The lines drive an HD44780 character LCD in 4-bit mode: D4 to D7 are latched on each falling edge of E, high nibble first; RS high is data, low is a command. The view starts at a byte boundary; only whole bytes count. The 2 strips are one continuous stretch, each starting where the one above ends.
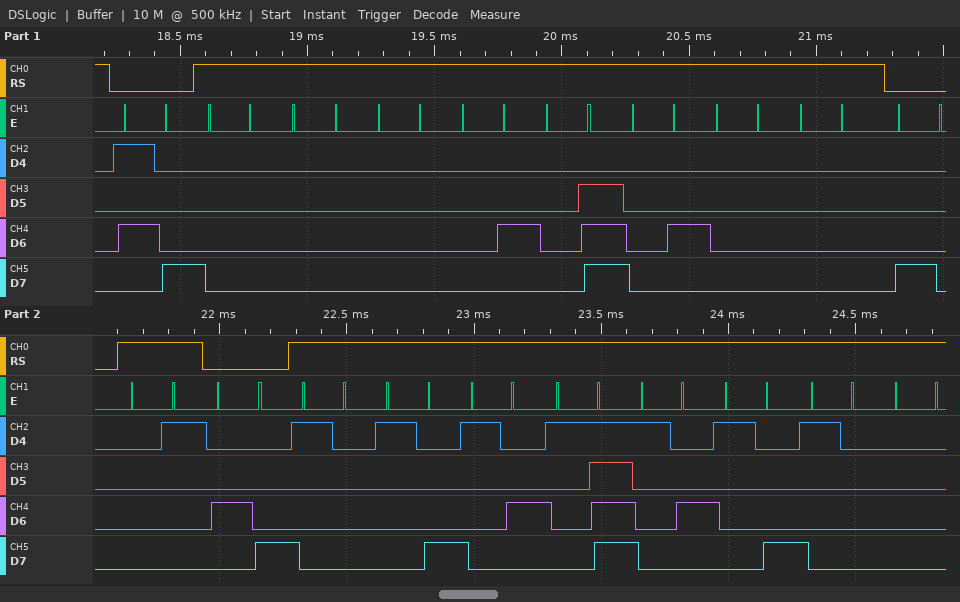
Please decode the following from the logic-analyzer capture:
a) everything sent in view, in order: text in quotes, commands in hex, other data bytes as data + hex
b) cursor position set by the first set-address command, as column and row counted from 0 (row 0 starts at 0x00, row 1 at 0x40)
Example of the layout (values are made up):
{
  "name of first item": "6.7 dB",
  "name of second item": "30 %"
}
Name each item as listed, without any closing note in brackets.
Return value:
{
  "everything sent in view, in order: text in quotes, commands in hex, other data bytes as data + hex": "0x58 data 00 00 00 04 0E 04 00 00 0x80 data 01 0x48 data 10 18 14 1F 14 18 10 00",
  "cursor position set by the first set-address command, as column and row counted from 0": "column 0, row 0"
}
